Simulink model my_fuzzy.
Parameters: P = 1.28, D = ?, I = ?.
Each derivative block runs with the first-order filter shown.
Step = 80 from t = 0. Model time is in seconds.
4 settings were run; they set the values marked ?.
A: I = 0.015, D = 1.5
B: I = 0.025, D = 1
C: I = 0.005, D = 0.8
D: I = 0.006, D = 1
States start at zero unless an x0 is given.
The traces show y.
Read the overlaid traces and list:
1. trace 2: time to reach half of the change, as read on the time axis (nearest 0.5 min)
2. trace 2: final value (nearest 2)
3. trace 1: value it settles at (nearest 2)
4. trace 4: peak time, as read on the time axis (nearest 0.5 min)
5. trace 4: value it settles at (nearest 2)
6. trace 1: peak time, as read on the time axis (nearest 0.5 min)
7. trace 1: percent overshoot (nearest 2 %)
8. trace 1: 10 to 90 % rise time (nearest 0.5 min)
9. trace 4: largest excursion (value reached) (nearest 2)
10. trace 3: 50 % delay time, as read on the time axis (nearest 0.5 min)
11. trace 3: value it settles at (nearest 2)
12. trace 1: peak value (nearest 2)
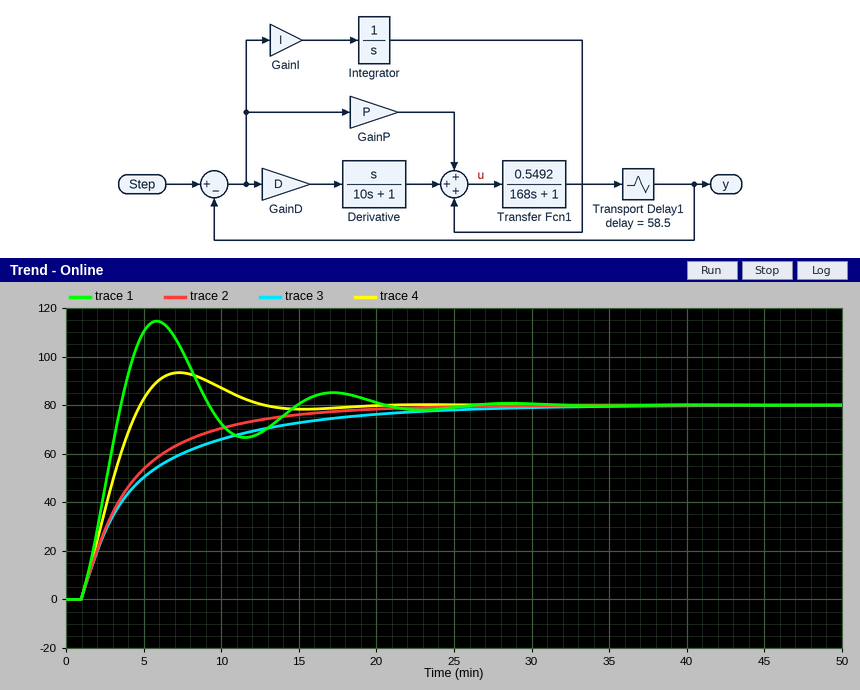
3.5 min
80
80
7.5 min
80
6.0 min
44 %
2.0 min
94
3.5 min
80
114
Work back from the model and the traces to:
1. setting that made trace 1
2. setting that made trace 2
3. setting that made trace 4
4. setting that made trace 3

B
D
A
C
